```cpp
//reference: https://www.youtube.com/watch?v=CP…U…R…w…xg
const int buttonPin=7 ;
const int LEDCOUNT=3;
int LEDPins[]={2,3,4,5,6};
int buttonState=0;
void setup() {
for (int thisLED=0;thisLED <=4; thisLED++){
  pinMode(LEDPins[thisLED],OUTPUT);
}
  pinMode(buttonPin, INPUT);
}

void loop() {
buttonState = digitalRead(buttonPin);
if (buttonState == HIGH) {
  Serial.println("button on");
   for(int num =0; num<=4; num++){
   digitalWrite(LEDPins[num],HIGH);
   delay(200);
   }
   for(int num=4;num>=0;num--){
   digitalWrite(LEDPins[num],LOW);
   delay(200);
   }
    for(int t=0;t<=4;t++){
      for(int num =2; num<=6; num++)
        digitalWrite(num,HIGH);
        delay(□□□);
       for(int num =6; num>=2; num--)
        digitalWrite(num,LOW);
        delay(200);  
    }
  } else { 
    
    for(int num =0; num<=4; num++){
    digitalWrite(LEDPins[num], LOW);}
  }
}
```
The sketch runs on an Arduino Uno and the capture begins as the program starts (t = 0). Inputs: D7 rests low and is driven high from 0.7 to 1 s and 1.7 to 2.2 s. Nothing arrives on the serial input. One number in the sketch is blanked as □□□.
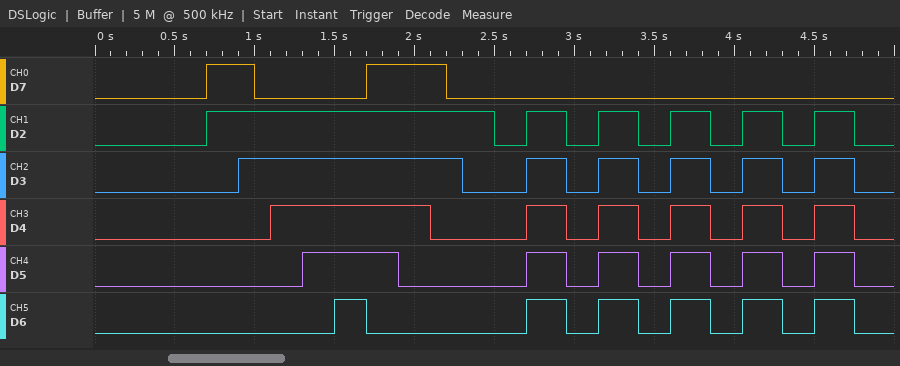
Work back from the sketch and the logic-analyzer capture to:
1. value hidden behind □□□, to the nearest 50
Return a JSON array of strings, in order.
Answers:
["250"]
